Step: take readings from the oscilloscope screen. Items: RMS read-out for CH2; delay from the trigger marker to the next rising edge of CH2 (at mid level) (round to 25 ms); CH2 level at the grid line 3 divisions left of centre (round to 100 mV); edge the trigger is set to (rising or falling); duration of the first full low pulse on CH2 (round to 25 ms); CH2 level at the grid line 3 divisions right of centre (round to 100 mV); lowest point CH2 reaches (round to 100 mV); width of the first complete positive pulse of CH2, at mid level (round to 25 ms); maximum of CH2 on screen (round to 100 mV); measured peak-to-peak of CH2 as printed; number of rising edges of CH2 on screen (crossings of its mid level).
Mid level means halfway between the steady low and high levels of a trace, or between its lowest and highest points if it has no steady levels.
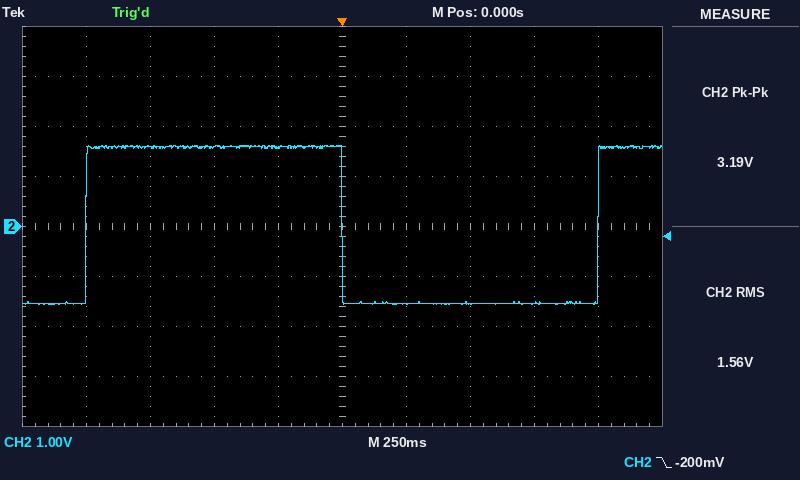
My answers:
1.56 V
1.000 s
1.6 V
falling
1.000 s
-1.5 V
-1.6 V
1.000 s
1.6 V
3.19 V
2
